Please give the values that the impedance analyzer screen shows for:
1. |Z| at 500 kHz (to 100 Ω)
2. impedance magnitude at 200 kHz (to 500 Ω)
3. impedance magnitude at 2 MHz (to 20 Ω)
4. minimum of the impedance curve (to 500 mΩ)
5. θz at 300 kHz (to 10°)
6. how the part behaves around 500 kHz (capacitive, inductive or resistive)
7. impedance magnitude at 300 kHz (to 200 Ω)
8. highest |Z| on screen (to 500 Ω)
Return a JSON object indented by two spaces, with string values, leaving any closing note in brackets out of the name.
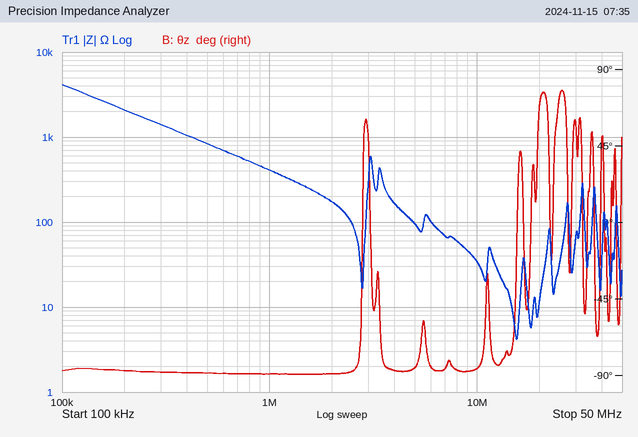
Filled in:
{
  "|Z| at 500 kHz": "800 Ω",
  "impedance magnitude at 200 kHz": "2.0 kΩ",
  "impedance magnitude at 2 MHz": "180 Ω",
  "minimum of the impedance curve": "4.0 Ω",
  "θz at 300 kHz": "-90°",
  "how the part behaves around 500 kHz": "capacitive",
  "impedance magnitude at 300 kHz": "1.4 kΩ",
  "highest |Z| on screen": "4.0 kΩ"
}
